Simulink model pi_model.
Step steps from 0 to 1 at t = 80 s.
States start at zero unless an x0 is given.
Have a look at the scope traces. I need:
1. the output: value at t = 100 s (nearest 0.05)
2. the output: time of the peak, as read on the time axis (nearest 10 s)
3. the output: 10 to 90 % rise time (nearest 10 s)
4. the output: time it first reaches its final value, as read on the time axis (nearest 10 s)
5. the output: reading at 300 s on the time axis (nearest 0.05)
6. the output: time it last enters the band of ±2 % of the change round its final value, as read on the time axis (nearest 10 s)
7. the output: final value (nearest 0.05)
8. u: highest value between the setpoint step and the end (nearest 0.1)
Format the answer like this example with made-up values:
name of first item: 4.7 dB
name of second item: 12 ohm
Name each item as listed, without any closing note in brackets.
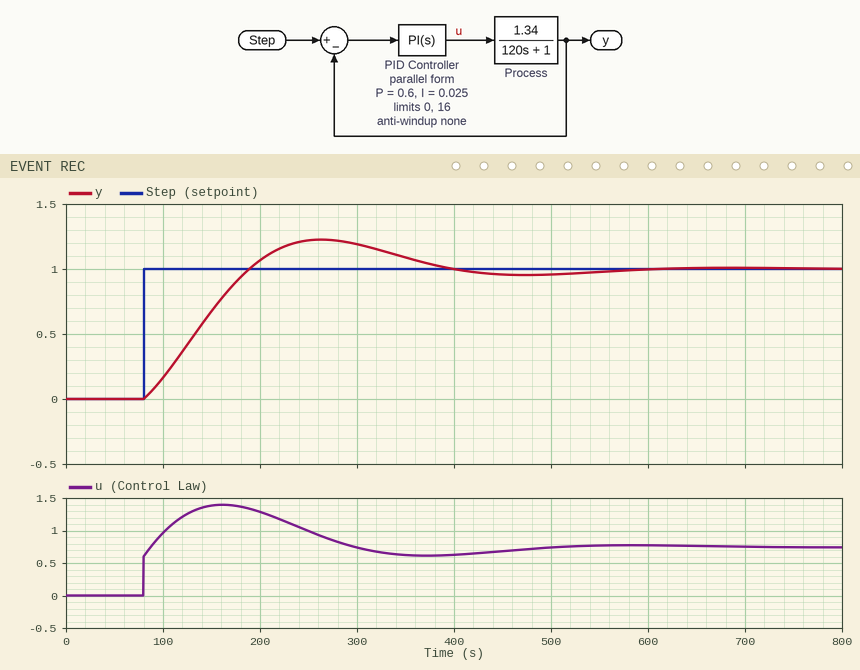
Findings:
the output: value at t = 100 s: 0.15
the output: time of the peak, as read on the time axis: 260 s
the output: 10 to 90 % rise time: 80 s
the output: time it first reaches its final value, as read on the time axis: 190 s
the output: reading at 300 s on the time axis: 1.20
the output: time it last enters the band of ±2 % of the change round its final value, as read on the time axis: 560 s
the output: final value: 1.00
u: highest value between the setpoint step and the end: 1.4
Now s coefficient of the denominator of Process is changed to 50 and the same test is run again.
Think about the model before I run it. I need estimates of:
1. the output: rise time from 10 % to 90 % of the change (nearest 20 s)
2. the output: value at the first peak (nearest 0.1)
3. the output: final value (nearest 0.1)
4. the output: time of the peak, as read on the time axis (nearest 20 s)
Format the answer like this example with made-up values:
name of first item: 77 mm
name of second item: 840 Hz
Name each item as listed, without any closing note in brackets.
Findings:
the output: rise time from 10 % to 90 % of the change: 60 s
the output: value at the first peak: 1.1
the output: final value: 1.0
the output: time of the peak, as read on the time axis: 220 s
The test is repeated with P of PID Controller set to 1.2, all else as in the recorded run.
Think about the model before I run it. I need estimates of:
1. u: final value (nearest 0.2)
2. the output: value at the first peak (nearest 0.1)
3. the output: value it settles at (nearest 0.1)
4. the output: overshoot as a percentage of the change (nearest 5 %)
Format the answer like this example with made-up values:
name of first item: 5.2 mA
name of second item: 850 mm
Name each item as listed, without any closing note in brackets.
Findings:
u: final value: 0.8
the output: value at the first peak: 1.1
the output: value it settles at: 1.0
the output: overshoot as a percentage of the change: 10 %
